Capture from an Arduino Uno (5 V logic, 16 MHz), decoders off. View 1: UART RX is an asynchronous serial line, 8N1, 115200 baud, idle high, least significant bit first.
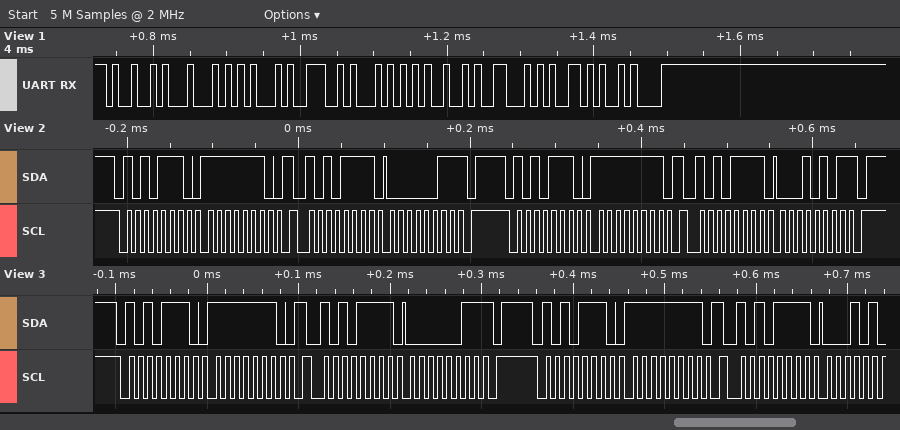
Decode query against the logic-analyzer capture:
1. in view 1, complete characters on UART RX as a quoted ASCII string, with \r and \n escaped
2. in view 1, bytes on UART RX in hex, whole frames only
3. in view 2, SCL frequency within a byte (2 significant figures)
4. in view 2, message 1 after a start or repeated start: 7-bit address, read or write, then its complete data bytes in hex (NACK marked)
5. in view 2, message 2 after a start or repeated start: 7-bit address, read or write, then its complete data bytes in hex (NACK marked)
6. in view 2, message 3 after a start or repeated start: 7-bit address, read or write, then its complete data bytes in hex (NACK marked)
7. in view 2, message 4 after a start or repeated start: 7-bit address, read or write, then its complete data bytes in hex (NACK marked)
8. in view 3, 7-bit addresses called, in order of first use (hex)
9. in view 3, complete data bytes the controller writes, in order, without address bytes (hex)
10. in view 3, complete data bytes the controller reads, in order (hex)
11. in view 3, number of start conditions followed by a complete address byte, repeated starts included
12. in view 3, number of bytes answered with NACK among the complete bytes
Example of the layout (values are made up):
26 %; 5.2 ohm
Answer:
"IDENTIFY\n"; 49 44 45 4E 54 49 46 59 0A; 100 kHz; 0x57 write: FE; 0x57 read: 03 NACK; 0x57 write: FF; 0x57 read: 15 NACK; 0x57; FE FF; 03; 4; 1
